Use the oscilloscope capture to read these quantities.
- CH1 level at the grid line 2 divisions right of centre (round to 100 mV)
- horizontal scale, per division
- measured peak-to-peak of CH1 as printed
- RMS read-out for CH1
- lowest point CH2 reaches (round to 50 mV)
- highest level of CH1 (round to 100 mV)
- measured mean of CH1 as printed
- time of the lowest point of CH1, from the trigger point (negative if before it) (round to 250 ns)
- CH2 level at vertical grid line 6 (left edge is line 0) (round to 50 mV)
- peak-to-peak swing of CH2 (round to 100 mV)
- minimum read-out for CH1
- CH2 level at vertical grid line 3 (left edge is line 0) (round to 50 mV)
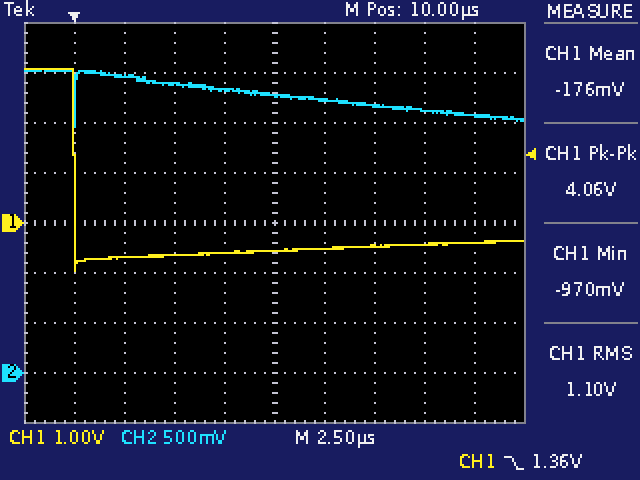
-500 mV
2.5 µs
4.06 V
1.10 V
2.45 V
3.1 V
-176 mV
0.00 µs
2.75 V
600 mV
-970 mV
2.90 V
